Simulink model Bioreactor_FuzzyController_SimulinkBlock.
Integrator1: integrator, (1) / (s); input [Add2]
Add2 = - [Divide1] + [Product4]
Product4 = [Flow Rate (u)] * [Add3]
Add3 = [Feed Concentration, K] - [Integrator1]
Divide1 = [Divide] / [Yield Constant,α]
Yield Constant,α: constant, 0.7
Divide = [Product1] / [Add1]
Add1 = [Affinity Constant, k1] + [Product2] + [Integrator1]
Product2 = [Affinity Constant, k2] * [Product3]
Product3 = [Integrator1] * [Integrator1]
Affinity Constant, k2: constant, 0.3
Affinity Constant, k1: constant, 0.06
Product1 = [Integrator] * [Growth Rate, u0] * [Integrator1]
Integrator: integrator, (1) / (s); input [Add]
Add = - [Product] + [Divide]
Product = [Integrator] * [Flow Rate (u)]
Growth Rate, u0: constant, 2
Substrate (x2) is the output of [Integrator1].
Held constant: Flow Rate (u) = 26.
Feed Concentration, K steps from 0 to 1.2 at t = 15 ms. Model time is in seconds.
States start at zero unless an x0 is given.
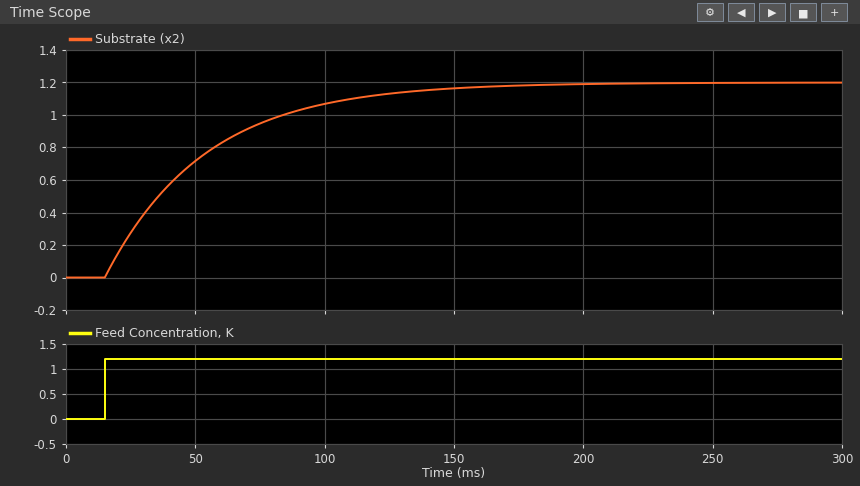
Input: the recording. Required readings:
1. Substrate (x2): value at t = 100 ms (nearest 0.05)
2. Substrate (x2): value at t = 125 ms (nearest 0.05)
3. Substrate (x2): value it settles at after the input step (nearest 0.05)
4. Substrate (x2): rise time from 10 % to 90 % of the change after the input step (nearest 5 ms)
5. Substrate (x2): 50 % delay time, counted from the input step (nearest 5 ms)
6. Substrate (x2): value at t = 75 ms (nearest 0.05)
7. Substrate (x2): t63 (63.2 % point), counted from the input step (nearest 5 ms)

1.05
1.15
1.20
85 ms
25 ms
0.95
40 ms
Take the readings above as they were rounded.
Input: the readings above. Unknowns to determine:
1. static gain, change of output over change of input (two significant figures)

1.0
